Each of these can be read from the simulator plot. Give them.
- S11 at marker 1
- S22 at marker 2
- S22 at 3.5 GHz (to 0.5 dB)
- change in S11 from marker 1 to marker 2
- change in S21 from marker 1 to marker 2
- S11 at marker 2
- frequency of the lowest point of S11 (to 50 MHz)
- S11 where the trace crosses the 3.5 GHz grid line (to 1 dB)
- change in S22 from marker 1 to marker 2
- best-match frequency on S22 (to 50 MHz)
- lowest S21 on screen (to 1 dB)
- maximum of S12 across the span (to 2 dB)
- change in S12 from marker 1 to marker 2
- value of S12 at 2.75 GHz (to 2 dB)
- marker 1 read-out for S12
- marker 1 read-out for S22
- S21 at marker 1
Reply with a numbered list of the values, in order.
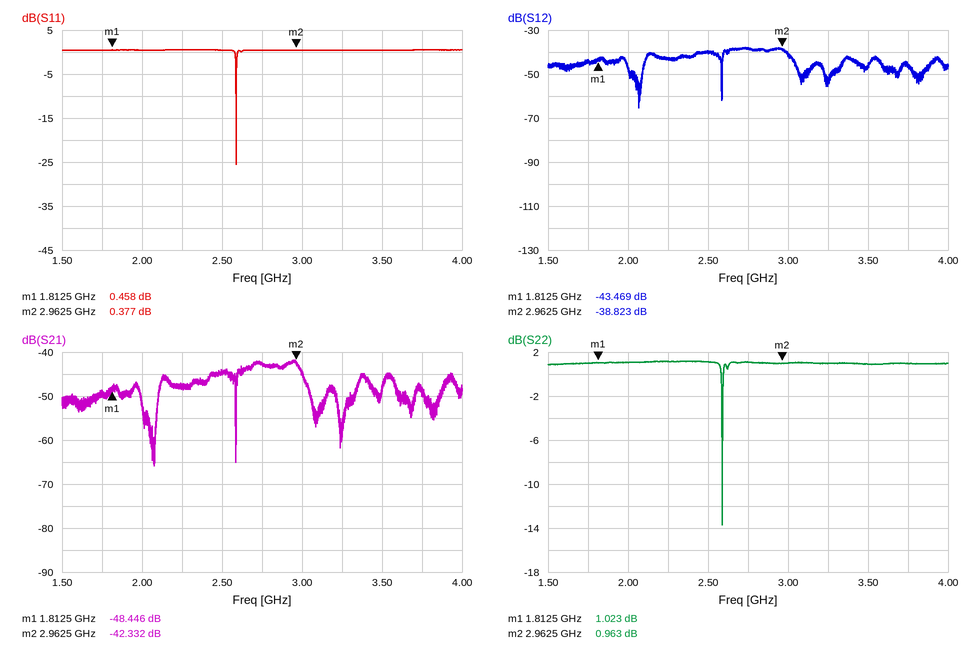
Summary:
1. 0.458 dB
2. 0.963 dB
3. 1.0 dB
4. -0.081 dB
5. 6.114 dB
6. 0.377 dB
7. 2.60 GHz
8. 0 dB
9. -0.060 dB
10. 2.60 GHz
11. -66 dB
12. -38 dB
13. 4.646 dB
14. -38 dB
15. -43.469 dB
16. 1.023 dB
17. -48.446 dB
